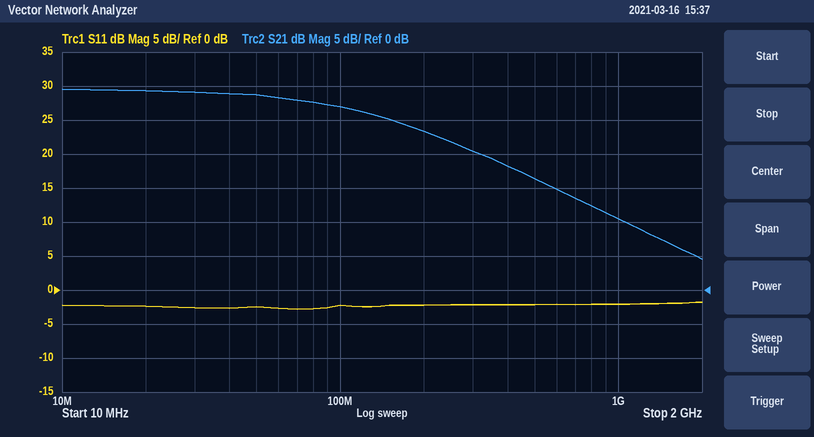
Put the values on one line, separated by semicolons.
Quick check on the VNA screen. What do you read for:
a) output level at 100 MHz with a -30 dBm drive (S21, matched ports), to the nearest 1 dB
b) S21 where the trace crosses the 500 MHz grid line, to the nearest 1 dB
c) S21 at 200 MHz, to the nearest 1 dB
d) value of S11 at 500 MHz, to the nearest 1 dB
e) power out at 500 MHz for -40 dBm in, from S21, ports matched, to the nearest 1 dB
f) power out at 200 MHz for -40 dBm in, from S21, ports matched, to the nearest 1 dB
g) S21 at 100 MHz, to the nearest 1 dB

-3 dBm; 16 dB; 23 dB; -2 dB; -24 dBm; -17 dBm; 27 dB
